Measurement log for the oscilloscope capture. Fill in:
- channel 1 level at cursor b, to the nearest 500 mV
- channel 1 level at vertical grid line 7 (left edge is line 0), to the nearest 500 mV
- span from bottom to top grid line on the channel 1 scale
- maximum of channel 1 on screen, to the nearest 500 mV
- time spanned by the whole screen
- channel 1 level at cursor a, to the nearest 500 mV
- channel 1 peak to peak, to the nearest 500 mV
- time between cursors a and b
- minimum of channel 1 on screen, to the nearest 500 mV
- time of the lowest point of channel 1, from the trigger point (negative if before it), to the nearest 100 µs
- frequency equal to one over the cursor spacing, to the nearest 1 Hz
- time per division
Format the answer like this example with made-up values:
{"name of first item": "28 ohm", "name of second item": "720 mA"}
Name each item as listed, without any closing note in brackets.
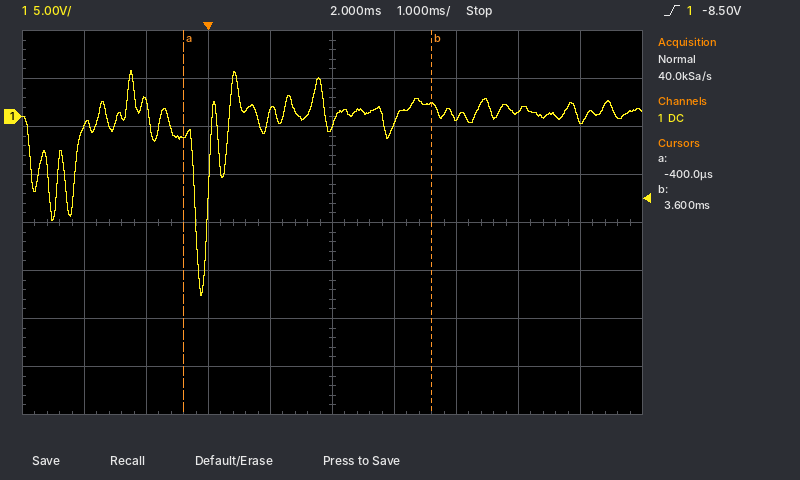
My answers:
{"channel 1 level at cursor b, to the nearest 500 mV": "1.5 V", "channel 1 level at vertical grid line 7 (left edge is line 0), to the nearest 500 mV": "0.0 V", "span from bottom to top grid line on the channel 1 scale": "40 V", "maximum of channel 1 on screen, to the nearest 500 mV": "5.0 V", "time spanned by the whole screen": "10 ms", "channel 1 level at cursor a, to the nearest 500 mV": "-2.0 V", "channel 1 peak to peak, to the nearest 500 mV": "23.5 V", "time between cursors a and b": "4.0 ms", "minimum of channel 1 on screen, to the nearest 500 mV": "-18.5 V", "time of the lowest point of channel 1, from the trigger point (negative if before it), to the nearest 100 µs": "-100 µs", "frequency equal to one over the cursor spacing, to the nearest 1 Hz": "250 Hz", "time per division": "1 ms"}
